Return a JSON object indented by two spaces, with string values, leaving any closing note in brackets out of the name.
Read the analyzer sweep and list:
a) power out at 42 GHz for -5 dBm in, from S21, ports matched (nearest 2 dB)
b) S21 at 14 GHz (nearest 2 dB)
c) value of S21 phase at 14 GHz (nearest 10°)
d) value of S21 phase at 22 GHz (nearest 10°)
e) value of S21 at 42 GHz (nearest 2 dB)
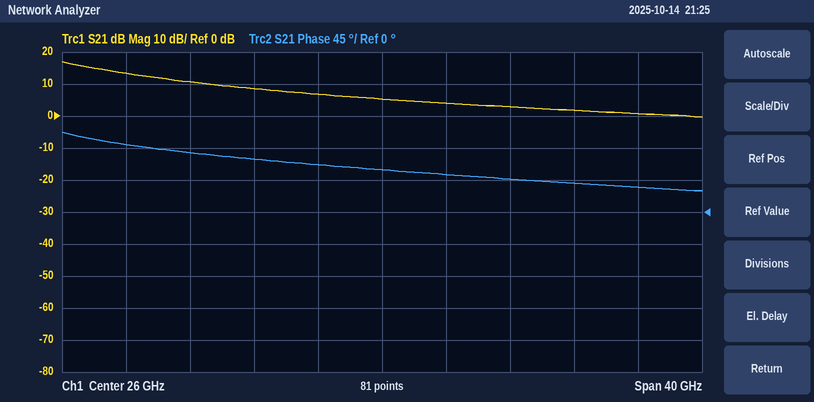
{
  "power out at 42 GHz for -5 dBm in, from S21, ports matched": "-4 dBm",
  "S21 at 14 GHz": "10 dB",
  "value of S21 phase at 14 GHz": "80°",
  "value of S21 phase at 22 GHz": "70°",
  "value of S21 at 42 GHz": "0 dB"
}
